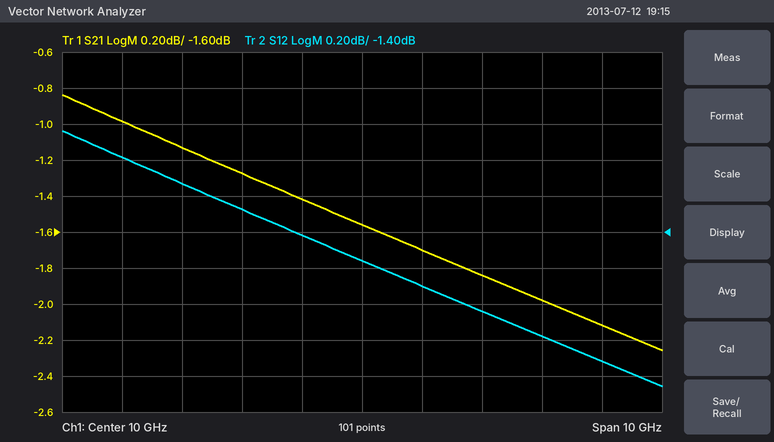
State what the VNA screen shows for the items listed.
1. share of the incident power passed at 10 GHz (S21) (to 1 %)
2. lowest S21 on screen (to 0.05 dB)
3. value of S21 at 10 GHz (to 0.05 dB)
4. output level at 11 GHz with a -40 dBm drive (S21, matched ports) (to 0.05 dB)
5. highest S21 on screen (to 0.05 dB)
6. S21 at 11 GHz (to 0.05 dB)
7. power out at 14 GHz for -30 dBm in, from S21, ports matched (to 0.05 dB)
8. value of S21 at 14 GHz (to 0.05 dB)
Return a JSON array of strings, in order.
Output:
["70 %", "-2.25 dB", "-1.55 dB", "-41.70 dBm", "-0.85 dB", "-1.70 dB", "-32.10 dBm", "-2.10 dB"]
